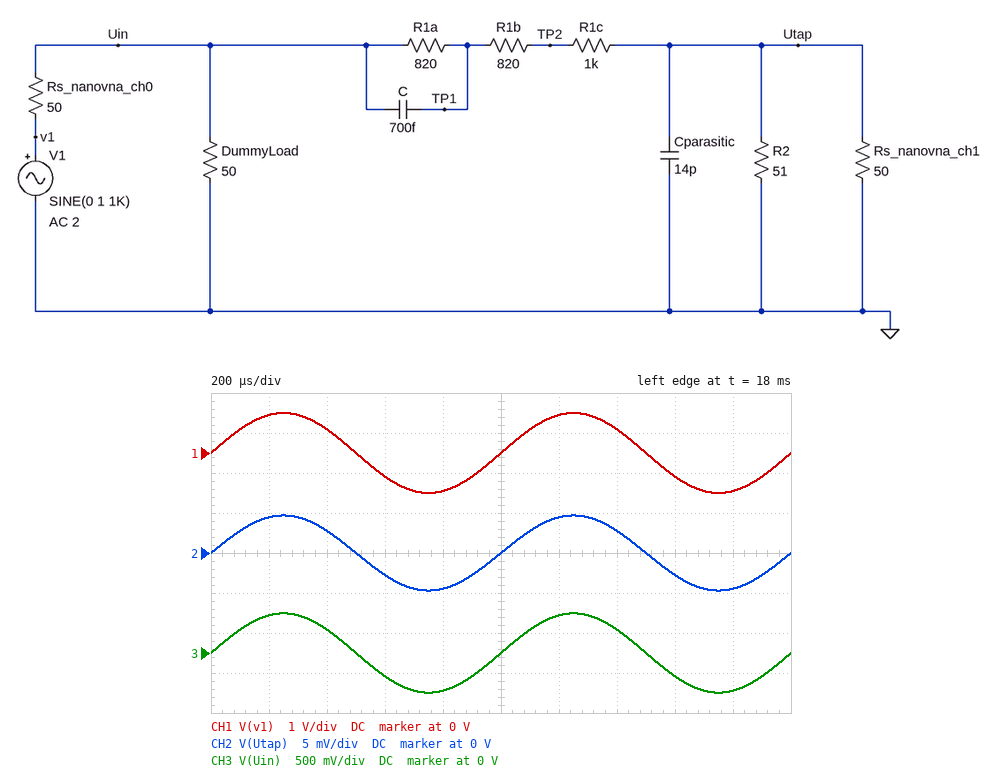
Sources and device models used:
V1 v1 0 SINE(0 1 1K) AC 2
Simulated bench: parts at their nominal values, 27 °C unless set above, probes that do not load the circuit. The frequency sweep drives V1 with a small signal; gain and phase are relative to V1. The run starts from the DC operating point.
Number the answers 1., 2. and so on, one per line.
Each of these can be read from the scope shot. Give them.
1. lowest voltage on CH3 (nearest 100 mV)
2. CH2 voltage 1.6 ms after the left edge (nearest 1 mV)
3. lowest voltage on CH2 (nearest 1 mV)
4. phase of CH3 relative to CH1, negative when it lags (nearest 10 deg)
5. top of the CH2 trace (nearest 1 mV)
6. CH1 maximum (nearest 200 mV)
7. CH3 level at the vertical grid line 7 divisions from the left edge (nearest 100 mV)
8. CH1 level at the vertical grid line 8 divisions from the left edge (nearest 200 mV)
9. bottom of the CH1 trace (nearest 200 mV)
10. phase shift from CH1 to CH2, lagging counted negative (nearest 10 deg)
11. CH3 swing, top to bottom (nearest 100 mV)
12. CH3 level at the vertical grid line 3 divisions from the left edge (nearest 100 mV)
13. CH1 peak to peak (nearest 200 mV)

1. -500 mV
2. -3 mV
3. -5 mV
4. 0 deg
5. 5 mV
6. 1.0 V
7. 300 mV
8. -600 mV
9. -1.0 V
10. 0 deg
11. 1.0 V
12. -300 mV
13. 2.0 V
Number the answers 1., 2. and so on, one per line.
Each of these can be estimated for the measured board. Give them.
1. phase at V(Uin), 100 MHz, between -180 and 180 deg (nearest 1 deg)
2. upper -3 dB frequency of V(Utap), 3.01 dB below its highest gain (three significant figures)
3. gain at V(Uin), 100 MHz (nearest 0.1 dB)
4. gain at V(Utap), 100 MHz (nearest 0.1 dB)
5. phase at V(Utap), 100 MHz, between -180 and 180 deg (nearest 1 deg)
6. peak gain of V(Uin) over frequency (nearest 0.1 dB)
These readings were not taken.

1. 0 deg
2. 731 MHz
3. -6.1 dB
4. -46.5 dB
5. -7 deg
6. -6.1 dB
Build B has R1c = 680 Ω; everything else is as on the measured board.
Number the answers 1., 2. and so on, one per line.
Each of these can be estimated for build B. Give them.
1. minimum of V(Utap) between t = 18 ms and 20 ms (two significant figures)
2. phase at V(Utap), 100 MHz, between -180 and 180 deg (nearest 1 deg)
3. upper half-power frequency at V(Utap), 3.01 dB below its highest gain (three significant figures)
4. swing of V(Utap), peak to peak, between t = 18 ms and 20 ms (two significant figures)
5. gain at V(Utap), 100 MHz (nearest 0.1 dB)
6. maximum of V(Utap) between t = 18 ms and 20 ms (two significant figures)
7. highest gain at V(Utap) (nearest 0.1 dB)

1. -5.3 mV
2. -6 deg
3. 778 MHz
4. 11 mV
5. -45.4 dB
6. 5.3 mV
7. -45.3 dB
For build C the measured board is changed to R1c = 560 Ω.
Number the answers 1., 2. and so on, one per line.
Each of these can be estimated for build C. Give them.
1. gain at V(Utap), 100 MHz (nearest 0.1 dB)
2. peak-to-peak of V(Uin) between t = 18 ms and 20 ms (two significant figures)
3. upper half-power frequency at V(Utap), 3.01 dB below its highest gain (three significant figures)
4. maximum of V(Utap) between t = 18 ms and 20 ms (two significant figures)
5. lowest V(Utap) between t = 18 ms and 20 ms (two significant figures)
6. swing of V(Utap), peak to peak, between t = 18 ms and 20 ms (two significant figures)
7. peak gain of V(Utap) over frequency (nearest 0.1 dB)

1. -44.9 dB
2. 990 mV
3. 800 MHz
4. 5.6 mV
5. -5.6 mV
6. 11 mV
7. -44.8 dB
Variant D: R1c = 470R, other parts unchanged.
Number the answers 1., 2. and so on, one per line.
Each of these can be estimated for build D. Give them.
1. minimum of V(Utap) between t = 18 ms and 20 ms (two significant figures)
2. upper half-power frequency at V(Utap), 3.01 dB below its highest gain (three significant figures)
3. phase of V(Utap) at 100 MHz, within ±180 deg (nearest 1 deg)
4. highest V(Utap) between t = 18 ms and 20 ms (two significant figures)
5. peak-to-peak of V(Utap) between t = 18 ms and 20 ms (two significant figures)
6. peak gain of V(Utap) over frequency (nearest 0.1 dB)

1. -5.8 mV
2. 818 MHz
3. -5 deg
4. 5.8 mV
5. 12 mV
6. -44.4 dB
